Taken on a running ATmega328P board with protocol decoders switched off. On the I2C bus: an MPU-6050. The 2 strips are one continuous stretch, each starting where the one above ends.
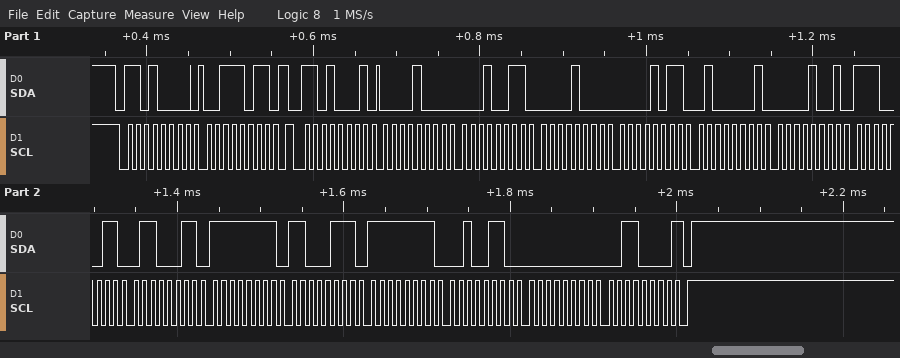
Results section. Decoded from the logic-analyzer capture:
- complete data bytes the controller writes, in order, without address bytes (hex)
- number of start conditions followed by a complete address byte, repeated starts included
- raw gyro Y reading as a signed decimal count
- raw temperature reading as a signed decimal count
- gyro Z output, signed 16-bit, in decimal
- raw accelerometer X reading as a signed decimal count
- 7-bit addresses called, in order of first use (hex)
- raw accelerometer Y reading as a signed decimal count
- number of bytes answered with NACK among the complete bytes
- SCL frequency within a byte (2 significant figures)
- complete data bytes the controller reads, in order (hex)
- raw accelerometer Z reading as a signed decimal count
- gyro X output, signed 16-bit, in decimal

3B
2
-218
-7325
48
2067
0x68
2059
1
100 kHz
08 13 08 0B 41 09 E3 63 FF C7 FF 26 00 30
16649
-57
